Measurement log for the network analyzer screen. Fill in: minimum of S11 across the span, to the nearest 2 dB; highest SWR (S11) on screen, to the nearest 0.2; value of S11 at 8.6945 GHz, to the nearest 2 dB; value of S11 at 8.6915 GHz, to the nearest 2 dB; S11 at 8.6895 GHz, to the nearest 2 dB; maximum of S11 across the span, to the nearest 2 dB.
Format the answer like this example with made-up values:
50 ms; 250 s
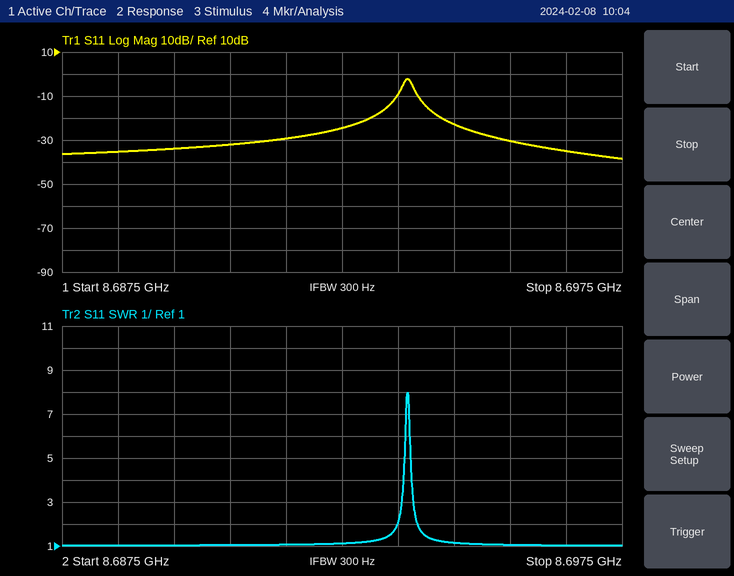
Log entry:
-38 dB; 8.0; -22 dB; -30 dB; -34 dB; -2 dB
